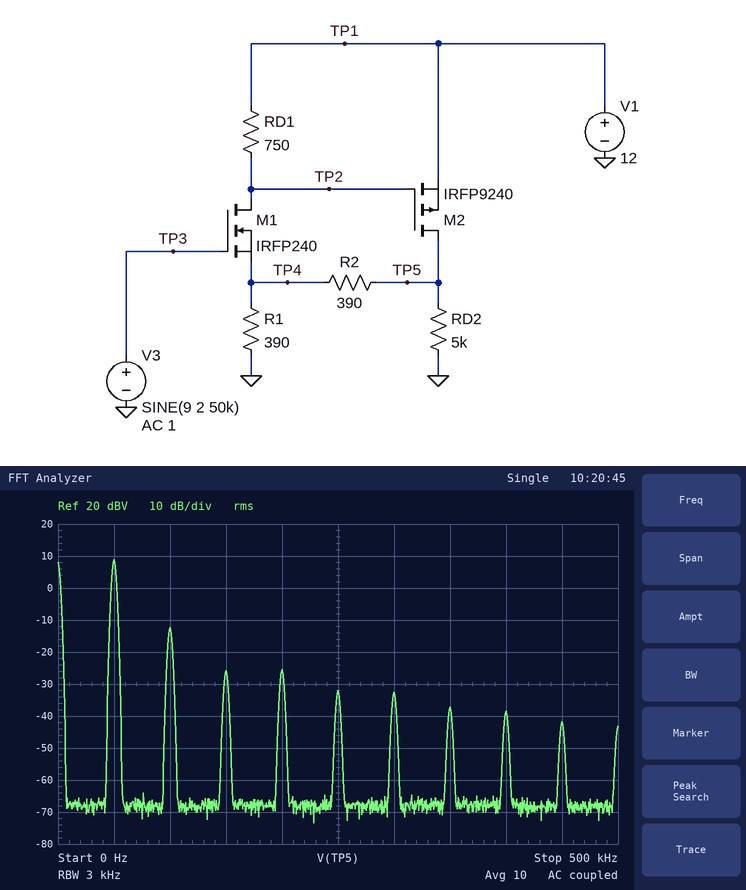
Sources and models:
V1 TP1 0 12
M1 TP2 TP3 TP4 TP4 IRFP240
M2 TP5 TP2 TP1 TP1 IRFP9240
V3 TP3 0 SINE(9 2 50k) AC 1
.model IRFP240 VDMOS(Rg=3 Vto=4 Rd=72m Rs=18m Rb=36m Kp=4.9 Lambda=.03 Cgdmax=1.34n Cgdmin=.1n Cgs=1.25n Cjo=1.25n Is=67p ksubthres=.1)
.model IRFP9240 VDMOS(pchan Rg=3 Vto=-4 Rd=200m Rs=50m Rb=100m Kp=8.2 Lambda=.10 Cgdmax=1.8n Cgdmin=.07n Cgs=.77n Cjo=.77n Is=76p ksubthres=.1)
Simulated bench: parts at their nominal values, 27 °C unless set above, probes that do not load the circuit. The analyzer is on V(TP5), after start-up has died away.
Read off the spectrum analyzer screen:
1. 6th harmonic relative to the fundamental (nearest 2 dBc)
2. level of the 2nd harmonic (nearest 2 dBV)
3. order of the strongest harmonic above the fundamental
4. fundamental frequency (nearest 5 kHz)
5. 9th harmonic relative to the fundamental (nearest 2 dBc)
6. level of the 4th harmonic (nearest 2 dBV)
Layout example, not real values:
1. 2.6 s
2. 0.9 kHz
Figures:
1. -42 dBc
2. -12 dBV
3. 2
4. 50 kHz
5. -50 dBc
6. -26 dBV
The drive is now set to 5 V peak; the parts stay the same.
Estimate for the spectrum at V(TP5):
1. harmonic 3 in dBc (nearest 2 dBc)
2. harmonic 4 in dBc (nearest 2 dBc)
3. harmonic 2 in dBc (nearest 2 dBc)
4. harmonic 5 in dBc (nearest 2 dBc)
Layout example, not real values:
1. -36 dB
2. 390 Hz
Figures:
1. -20 dBc
2. -22 dBc
3. -10 dBc
4. -26 dBc
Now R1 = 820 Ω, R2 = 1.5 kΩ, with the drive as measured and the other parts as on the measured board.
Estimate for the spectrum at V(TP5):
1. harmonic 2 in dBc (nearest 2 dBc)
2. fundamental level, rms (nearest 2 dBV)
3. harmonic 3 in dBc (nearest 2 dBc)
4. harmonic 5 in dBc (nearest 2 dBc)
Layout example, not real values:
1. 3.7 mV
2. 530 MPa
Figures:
1. -16 dBc
2. 10 dBV
3. -22 dBc
4. -30 dBc
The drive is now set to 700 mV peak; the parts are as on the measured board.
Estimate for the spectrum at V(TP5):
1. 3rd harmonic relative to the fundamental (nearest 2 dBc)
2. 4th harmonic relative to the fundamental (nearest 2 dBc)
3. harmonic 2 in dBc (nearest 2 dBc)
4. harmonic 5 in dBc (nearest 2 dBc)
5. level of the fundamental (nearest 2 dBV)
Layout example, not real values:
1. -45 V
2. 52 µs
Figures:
1. -42 dBc
2. -46 dBc
3. -26 dBc
4. -56 dBc
5. 0 dBV
